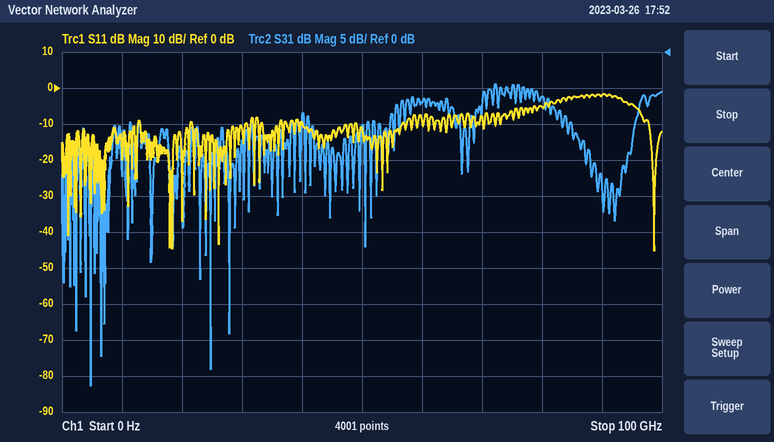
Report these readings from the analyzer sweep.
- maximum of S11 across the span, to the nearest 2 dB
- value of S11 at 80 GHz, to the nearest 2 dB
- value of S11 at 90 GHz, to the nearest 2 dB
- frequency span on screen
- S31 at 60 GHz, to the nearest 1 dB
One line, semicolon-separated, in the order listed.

-2 dB; -6 dB; -2 dB; 100 GHz; -7 dB
